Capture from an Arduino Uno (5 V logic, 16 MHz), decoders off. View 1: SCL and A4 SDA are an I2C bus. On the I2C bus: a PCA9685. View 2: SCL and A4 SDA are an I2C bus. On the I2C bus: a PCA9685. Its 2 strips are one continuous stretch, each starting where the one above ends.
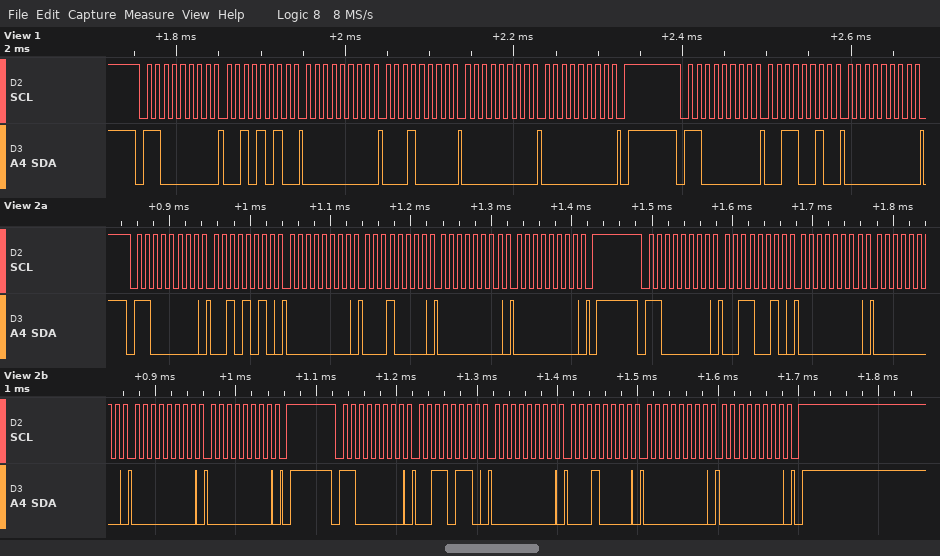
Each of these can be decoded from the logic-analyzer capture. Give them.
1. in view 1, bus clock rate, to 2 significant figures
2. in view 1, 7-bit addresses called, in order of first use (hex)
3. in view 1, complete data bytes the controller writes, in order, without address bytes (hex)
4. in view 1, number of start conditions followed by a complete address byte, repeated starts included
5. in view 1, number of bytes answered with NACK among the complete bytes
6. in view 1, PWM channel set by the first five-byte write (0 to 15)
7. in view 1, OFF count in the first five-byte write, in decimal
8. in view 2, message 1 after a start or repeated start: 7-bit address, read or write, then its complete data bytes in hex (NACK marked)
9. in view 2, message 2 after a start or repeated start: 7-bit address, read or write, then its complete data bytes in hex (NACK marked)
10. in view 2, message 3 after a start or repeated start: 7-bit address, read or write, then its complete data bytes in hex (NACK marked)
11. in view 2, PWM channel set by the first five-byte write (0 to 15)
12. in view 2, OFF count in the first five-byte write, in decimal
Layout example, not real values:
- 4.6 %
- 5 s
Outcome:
- 100 kHz
- 0x60
- 2A 00 10 00 00 32 00
- 2
- 0
- 9
- 0
- 0x60 write: 2A 00 10 00 00
- 0x60 write: 32 00 00 00 00
- 0x60 write: 36 00 10 00 00
- 9
- 0
